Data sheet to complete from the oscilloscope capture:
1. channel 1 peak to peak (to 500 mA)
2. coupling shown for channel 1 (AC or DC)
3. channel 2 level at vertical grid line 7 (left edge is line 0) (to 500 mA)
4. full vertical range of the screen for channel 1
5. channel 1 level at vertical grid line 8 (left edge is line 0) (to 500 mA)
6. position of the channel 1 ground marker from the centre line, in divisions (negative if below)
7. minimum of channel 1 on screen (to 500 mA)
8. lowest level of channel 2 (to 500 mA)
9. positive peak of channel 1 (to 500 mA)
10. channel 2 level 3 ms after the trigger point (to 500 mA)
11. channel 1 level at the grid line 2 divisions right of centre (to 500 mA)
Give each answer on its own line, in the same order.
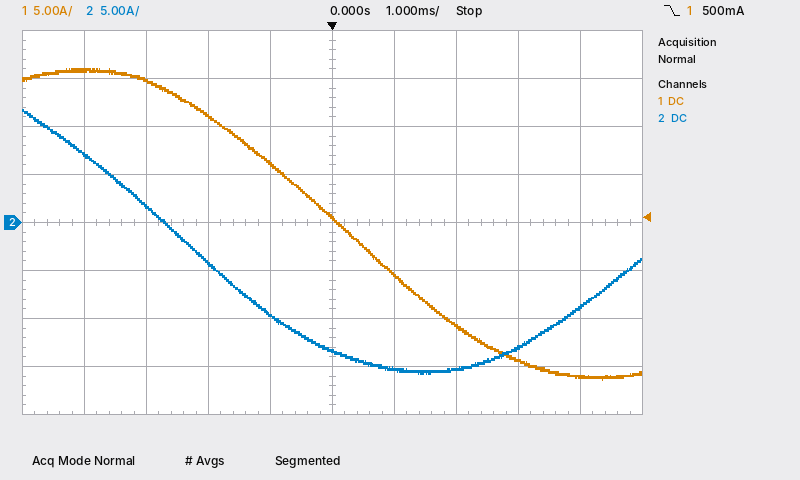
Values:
32.5 A
DC
-15.5 A
40 A
-14.5 A
0.0 div
-16.5 A
-16.0 A
16.0 A
-13.0 A
-11.0 A
